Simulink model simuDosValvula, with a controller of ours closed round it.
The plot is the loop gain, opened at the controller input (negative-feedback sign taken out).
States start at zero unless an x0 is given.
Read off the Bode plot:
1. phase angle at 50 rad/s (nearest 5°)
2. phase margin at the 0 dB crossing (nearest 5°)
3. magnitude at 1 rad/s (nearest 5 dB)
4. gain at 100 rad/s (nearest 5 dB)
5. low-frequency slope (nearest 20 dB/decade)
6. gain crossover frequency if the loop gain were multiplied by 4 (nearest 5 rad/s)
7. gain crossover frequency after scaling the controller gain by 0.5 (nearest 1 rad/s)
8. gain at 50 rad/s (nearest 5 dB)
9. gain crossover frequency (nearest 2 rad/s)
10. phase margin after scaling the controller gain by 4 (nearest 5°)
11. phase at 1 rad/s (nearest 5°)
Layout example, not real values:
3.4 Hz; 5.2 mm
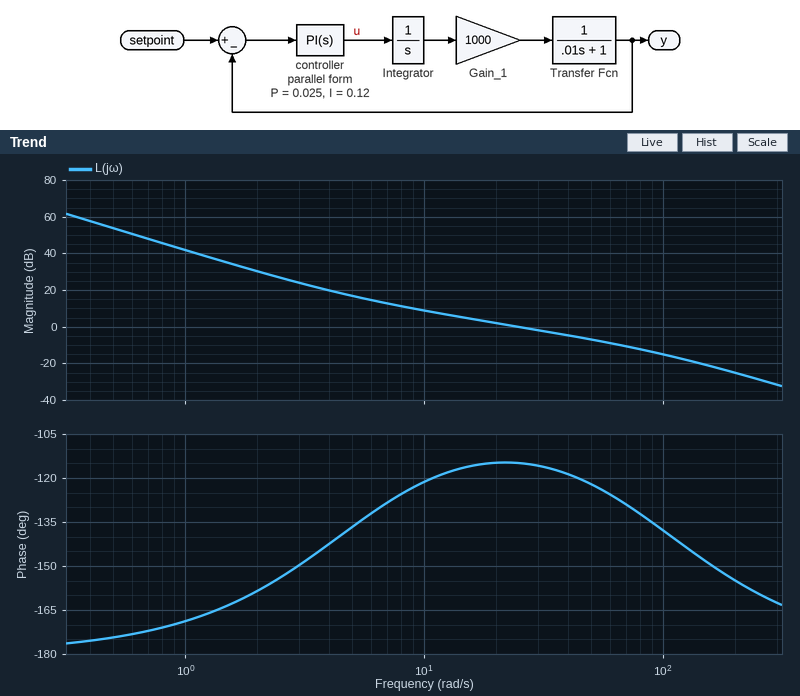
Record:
-120°; 65°; 40 dB; -15 dB; -40 dB/decade; 80 rad/s; 13 rad/s; -5 dB; 24 rad/s; 50°; -170°
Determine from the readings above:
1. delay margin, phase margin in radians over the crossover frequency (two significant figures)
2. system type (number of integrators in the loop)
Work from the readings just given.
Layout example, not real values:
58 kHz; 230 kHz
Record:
0.047 s; 2
